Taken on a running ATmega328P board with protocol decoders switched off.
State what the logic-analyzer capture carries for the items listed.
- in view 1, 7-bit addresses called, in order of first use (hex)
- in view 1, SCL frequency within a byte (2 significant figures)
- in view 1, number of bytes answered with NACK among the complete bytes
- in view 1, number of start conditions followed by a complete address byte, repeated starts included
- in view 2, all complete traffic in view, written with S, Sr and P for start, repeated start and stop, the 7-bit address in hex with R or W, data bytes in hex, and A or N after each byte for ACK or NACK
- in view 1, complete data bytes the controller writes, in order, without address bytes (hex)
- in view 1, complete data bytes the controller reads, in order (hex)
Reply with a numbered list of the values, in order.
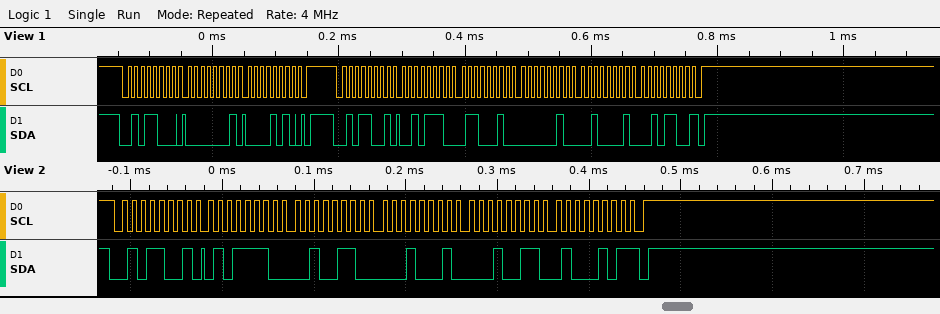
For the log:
1. 0x2C
2. 100 kHz
3. 1
4. 2
5. S 2CR A 5E A 26 A 11 A 13 A 45 N P
6. 01 0A
7. 2E 62 02 21 2C
